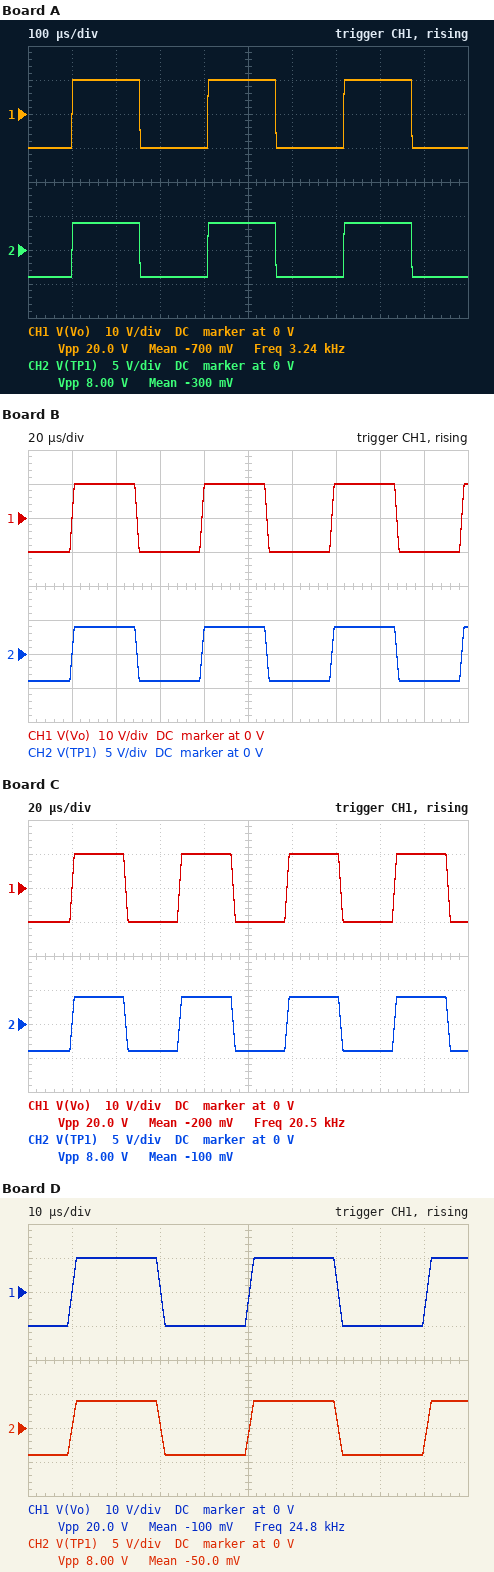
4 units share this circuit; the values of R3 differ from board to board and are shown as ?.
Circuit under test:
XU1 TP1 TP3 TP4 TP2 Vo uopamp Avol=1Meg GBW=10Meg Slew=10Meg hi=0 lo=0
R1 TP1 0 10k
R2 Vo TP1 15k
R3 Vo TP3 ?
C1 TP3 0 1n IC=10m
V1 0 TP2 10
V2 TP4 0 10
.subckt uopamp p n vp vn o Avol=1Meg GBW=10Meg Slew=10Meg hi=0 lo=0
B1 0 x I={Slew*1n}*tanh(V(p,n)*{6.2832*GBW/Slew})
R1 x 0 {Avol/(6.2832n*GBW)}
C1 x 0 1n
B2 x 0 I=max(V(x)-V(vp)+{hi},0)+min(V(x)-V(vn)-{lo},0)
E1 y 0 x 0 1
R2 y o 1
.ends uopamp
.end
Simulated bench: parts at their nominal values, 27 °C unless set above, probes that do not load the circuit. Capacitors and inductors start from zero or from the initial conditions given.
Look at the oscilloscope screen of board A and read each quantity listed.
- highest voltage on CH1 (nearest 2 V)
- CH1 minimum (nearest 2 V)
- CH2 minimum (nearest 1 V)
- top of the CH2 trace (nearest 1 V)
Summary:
10 V
-10 V
-4 V
4 V
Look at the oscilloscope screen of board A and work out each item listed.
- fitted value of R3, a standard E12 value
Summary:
180 kΩ
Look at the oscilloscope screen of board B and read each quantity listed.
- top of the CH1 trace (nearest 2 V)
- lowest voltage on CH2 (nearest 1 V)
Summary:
10 V
-4 V
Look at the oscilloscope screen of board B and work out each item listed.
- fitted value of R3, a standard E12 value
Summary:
33 kΩ
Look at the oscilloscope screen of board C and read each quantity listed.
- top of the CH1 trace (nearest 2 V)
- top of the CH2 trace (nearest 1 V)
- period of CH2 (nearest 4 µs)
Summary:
10 V
4 V
48 µs
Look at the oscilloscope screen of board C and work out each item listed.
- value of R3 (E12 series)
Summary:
27 kΩ
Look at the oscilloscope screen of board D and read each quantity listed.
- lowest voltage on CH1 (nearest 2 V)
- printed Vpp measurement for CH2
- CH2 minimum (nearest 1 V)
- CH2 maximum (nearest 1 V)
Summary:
-10 V
8.00 V
-4 V
4 V
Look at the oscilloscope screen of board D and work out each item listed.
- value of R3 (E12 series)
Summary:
22 kΩ
